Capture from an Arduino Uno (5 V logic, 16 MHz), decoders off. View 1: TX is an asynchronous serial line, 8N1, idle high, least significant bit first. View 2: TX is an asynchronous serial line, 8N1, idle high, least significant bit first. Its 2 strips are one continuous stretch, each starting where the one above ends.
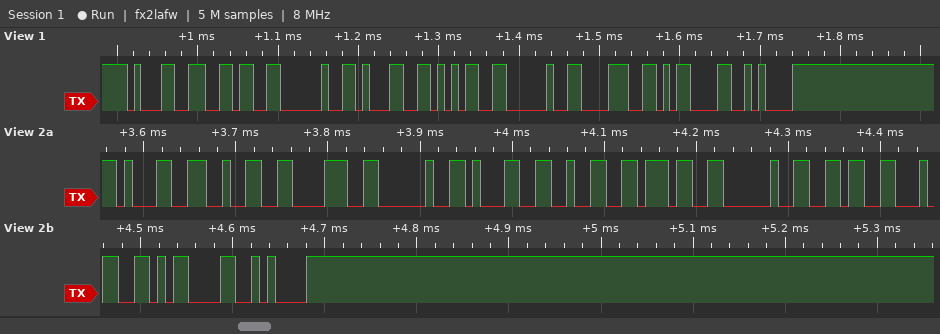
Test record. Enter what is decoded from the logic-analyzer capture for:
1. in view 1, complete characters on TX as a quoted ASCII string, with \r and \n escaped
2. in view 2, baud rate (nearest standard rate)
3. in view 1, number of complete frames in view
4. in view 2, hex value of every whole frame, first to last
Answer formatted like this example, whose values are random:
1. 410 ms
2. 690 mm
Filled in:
1. "16 15 8\r\n"
2. 115200 baud
3. 9
4. 0x31 0x32 0x38 0x20 0x31 0x32 0x37 0x20 0x36 0x34 0x0D 0x0A
